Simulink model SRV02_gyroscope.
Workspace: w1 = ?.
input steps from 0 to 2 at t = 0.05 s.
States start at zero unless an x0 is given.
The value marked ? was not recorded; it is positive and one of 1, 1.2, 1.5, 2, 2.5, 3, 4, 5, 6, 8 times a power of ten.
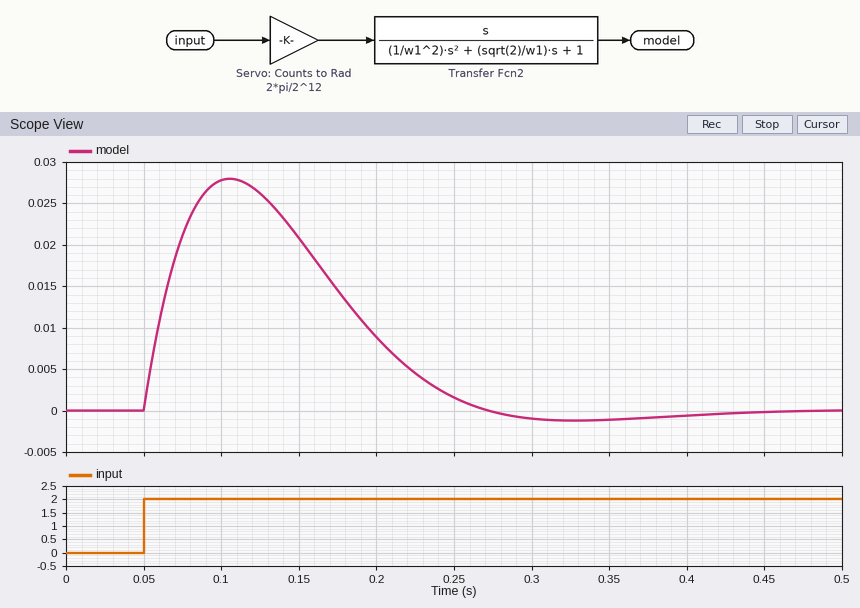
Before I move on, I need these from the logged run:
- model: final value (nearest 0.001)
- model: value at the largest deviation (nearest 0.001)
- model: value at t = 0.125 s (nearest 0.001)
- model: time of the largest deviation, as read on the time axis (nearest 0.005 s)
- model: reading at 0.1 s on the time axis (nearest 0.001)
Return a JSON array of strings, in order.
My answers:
["0.000", "0.028", "0.026", "0.105 s", "0.028"]
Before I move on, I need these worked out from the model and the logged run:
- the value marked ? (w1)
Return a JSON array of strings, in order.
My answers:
["20"]
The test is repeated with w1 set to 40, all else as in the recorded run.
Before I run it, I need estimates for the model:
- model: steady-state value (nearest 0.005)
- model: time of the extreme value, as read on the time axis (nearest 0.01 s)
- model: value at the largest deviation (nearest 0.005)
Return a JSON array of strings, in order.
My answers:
["0.000", "0.08 s", "0.055"]
